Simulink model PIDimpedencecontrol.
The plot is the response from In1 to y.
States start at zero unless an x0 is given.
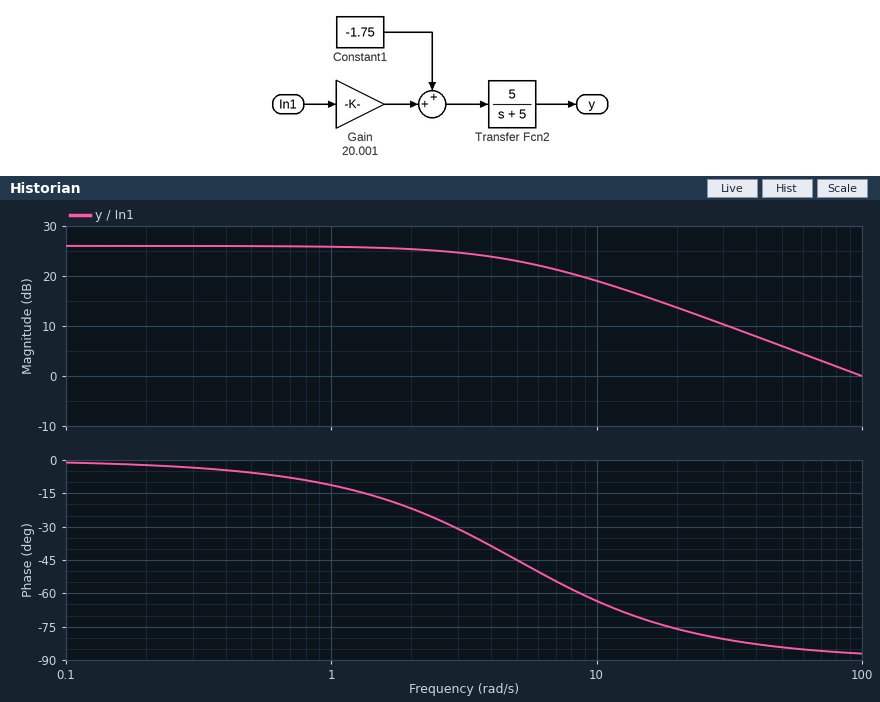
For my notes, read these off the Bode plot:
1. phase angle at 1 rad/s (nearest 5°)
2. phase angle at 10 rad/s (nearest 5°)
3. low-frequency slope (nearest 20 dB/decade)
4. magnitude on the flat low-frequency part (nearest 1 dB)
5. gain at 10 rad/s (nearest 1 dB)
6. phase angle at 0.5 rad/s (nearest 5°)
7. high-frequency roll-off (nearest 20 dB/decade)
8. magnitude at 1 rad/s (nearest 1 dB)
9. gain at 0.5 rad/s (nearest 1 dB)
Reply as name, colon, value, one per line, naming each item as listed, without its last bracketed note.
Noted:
phase angle at 1 rad/s: -10°
phase angle at 10 rad/s: -65°
low-frequency slope: 0 dB/decade
magnitude on the flat low-frequency part: 26 dB
gain at 10 rad/s: 19 dB
phase angle at 0.5 rad/s: -5°
high-frequency roll-off: -20 dB/decade
magnitude at 1 rad/s: 26 dB
gain at 0.5 rad/s: 26 dB
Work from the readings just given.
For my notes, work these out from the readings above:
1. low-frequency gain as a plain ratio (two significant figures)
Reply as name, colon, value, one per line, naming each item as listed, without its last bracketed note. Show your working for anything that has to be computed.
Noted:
low-frequency gain as a plain ratio: 10^(26 / 20) = 20
